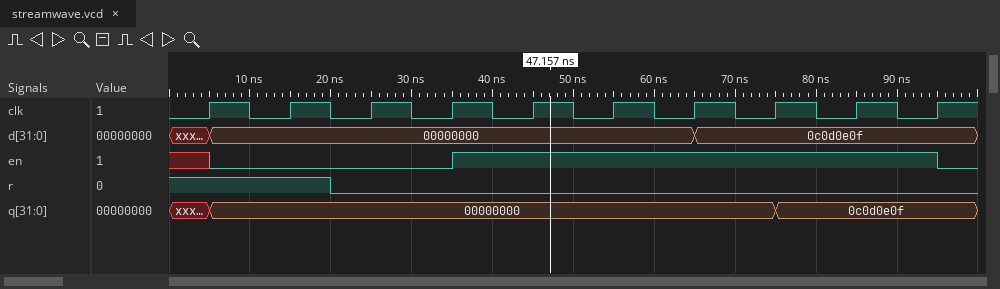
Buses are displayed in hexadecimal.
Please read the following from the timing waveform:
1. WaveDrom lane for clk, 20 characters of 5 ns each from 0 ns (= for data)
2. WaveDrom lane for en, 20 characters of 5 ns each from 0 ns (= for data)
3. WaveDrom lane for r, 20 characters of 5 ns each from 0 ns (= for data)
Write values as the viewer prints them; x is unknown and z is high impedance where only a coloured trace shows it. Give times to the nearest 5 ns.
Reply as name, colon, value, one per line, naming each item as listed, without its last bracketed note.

WaveDrom lane for clk, 20 characters of 5 ns each from 0 ns: {name: 'clk', wave: '01010101010101010101'}
WaveDrom lane for en, 20 characters of 5 ns each from 0 ns: {name: 'en', wave: 'x0.....1...........0'}
WaveDrom lane for r, 20 characters of 5 ns each from 0 ns: {name: 'r', wave: '1...0...............'}
